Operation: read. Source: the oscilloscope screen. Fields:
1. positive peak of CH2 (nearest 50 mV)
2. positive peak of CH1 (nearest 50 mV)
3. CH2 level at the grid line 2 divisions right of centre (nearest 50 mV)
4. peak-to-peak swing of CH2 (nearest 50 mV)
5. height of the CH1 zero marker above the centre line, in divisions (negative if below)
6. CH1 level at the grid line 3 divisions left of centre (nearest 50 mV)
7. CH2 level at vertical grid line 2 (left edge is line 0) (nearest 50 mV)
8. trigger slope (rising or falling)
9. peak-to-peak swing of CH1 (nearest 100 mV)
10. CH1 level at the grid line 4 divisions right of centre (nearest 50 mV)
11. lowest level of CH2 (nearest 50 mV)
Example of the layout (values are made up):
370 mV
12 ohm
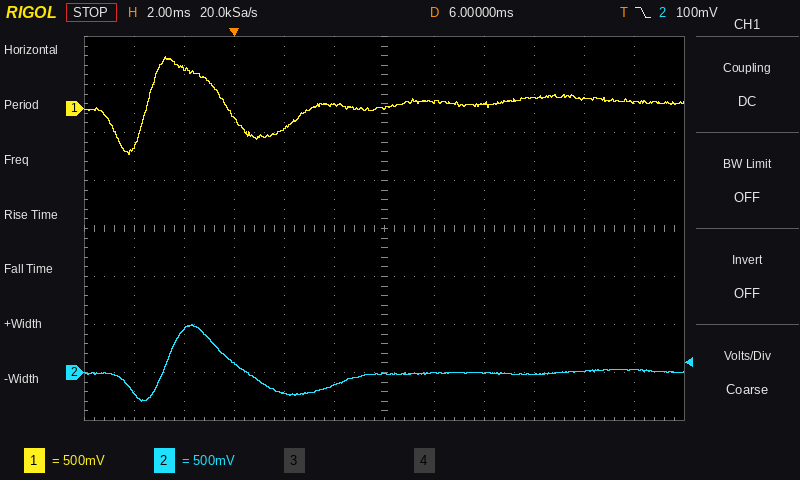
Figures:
500 mV
550 mV
0 mV
800 mV
+2.5 div
-100 mV
450 mV
falling
1.00 V
100 mV
-300 mV
